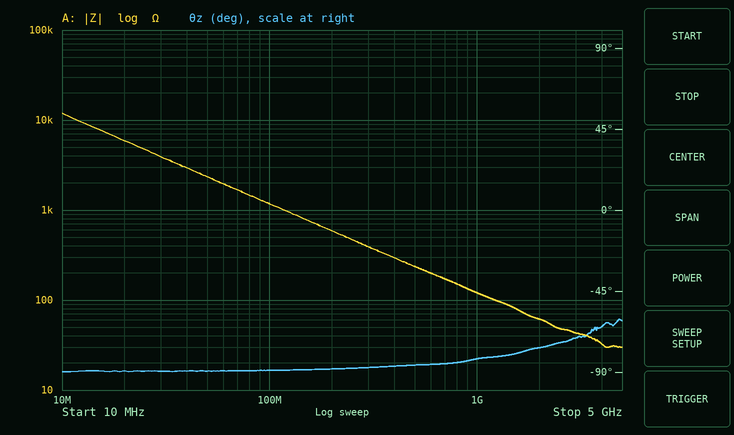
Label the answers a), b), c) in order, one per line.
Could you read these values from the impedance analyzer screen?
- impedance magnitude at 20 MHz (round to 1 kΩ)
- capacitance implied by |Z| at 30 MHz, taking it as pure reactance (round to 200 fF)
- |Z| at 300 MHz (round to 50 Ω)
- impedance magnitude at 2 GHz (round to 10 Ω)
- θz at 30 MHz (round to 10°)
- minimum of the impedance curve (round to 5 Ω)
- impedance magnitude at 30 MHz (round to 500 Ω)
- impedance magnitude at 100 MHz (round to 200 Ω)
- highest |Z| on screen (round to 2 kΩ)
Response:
a) 6 kΩ
b) 1.4 pF
c) 400 Ω
d) 60 Ω
e) -90°
f) 30 Ω
g) 4.0 kΩ
h) 1.2 kΩ
i) 12 kΩ
